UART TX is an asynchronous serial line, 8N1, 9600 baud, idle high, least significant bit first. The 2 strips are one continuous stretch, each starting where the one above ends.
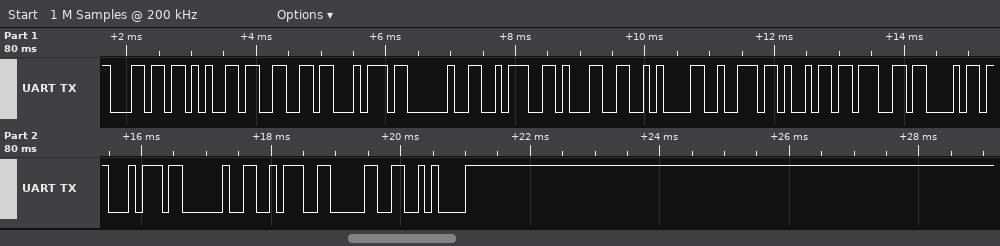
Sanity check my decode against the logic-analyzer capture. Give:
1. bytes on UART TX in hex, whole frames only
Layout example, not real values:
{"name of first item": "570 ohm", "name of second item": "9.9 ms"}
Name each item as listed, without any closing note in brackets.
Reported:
{"bytes on UART TX in hex, whole frames only": "0x6C 0x65 0x66 0x74 0x20 0x3A 0x31 0x0A 0x72 0x69 0x67 0x68 0x74 0x20 0x3A 0x30 0x0A"}
